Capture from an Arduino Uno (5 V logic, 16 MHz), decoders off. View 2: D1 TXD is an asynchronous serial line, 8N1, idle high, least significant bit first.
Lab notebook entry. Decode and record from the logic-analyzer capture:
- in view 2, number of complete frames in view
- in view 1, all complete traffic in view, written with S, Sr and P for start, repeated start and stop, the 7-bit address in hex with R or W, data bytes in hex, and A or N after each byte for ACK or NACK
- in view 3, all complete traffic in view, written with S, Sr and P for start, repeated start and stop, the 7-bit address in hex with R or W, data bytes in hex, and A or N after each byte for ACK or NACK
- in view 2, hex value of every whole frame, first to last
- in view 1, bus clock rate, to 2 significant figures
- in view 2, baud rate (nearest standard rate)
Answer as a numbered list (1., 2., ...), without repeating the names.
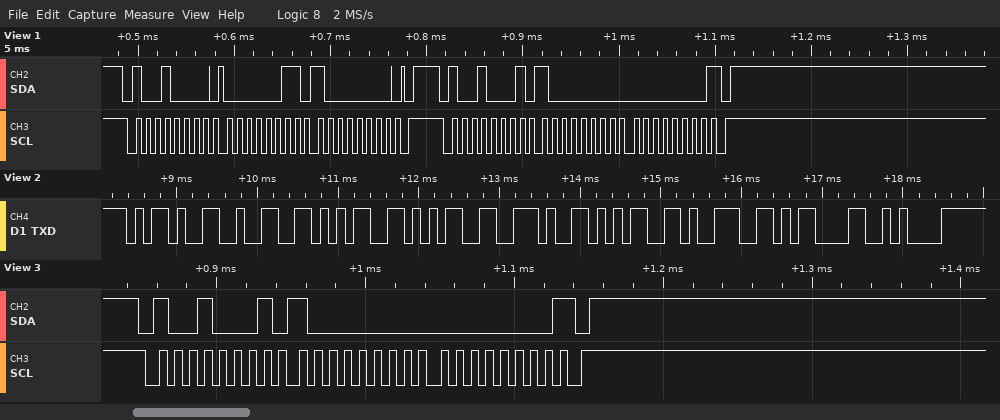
1. 9
2. S 48W A 03 A 80 A P S 48R A 80 A 00 N P
3. S 48R A 80 A 00 N P
4. 2D 32 35 35 2E 35 39 0D 0A
5. 100 kHz
6. 9600 baud
